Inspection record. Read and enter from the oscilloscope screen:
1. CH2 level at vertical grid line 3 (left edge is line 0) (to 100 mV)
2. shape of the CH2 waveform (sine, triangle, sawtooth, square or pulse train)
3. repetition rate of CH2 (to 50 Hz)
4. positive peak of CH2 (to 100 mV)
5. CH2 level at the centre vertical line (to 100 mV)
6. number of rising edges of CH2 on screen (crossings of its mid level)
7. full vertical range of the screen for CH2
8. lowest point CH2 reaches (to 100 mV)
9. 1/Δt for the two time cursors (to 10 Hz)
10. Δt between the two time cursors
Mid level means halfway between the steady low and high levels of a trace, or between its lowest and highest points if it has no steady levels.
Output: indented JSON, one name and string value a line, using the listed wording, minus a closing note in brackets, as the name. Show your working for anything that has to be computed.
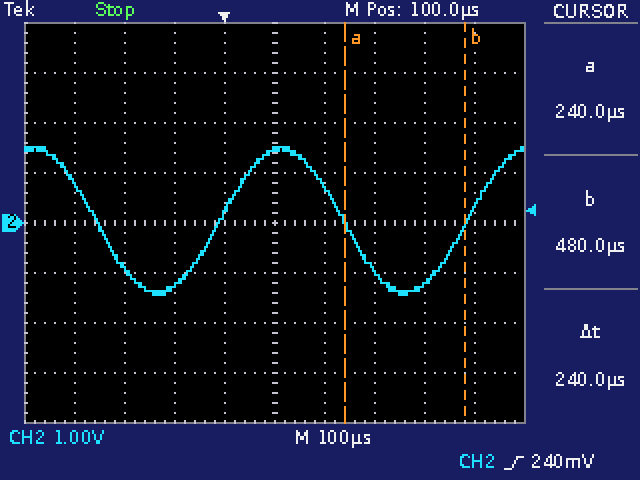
{
  "CH2 level at vertical grid line 3 (left edge is line 0)": "-1.3 V",
  "shape of the CH2 waveform": "sine",
  "repetition rate of CH2": "2.00 kHz",
  "positive peak of CH2": "1.5 V",
  "CH2 level at the centre vertical line": "1.5 V",
  "number of rising edges of CH2 on screen": "2",
  "full vertical range of the screen for CH2": "8 V",
  "lowest point CH2 reaches": "-1.4 V",
  "1/Δt for the two time cursors": "1 / 240 µs ≈ 4.17 kHz",
  "Δt between the two time cursors": "240 µs"
}
